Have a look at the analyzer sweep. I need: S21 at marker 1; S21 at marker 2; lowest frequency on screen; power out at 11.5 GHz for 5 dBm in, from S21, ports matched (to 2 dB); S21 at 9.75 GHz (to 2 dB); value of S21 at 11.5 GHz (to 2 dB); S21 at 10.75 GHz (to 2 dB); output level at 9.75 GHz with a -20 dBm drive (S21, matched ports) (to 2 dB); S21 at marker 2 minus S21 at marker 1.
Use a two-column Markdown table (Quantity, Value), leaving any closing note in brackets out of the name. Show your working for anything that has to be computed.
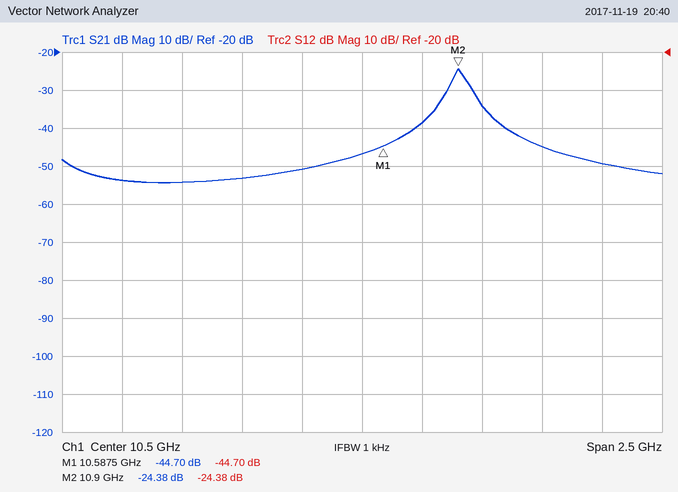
| Quantity | Value |
|---|---|
| S21 at marker 1 | -44.70 dB |
| S21 at marker 2 | -24.38 dB |
| lowest frequency on screen | 9.25 GHz |
| power out at 11.5 GHz for 5 dBm in, from S21, ports matched | 5 dBm + (-50 dB) = -44 dBm |
| S21 at 9.75 GHz | -54 dB |
| value of S21 at 11.5 GHz | -50 dB |
| S21 at 10.75 GHz | -38 dB |
| output level at 9.75 GHz with a -20 dBm drive (S21, matched ports) | -20 dBm + (-54 dB) = -74 dBm |
| S21 at marker 2 minus S21 at marker 1 | -24.38 − (-44.7) = 20.32 dB |
